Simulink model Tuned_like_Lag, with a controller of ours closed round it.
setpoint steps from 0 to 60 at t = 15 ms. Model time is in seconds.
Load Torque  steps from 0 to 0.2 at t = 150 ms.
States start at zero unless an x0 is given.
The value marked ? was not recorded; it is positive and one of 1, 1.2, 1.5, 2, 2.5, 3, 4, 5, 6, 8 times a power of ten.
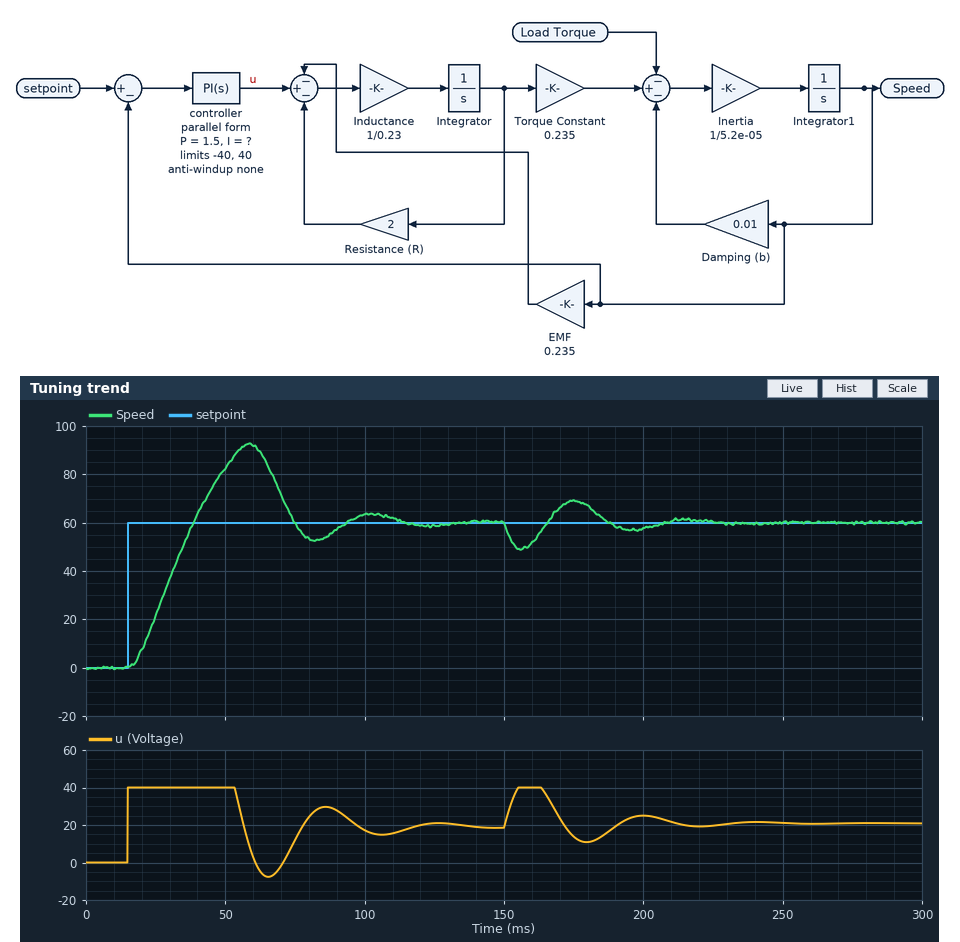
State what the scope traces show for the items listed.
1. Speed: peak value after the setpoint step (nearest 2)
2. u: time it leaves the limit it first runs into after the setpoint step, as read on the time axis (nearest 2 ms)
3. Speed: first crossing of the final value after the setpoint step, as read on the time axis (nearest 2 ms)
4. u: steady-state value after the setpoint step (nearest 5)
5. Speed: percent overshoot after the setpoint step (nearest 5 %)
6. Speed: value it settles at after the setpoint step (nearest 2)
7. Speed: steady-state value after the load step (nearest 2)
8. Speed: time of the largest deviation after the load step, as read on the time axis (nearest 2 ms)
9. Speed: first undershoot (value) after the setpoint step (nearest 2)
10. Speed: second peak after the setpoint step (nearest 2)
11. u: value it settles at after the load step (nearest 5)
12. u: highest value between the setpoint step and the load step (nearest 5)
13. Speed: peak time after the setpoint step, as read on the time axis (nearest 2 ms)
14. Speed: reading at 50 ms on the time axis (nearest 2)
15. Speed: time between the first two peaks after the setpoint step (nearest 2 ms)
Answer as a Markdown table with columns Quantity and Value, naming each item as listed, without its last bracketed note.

| Quantity | Value |
|---|---|
| Speed: peak value after the setpoint step | 92 |
| u: time it leaves the limit it first runs into after the setpoint step, as read on the time axis | 54 ms |
| Speed: first crossing of the final value after the setpoint step, as read on the time axis | 38 ms |
| u: steady-state value after the setpoint step | 20 |
| Speed: percent overshoot after the setpoint step | 55 % |
| Speed: value it settles at after the setpoint step | 60 |
| Speed: steady-state value after the load step | 60 |
| Speed: time of the largest deviation after the load step, as read on the time axis | 156 ms |
| Speed: first undershoot (value) after the setpoint step | 52 |
| Speed: second peak after the setpoint step | 64 |
| u: value it settles at after the load step | 20 |
| u: highest value between the setpoint step and the load step | 40 |
| Speed: peak time after the setpoint step, as read on the time axis | 58 ms |
| Speed: reading at 50 ms on the time axis | 82 |
| Speed: time between the first two peaks after the setpoint step | 44 ms |
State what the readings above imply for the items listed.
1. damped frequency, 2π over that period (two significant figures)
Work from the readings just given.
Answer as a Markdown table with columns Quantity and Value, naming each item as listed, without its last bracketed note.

| Quantity | Value |
|---|---|
| damped frequency, 2π over that period | 0.14 rad/ms |
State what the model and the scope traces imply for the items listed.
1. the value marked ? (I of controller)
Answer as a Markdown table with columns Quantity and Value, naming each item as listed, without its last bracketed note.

| Quantity | Value |
|---|---|
| the value marked ? | 150 |
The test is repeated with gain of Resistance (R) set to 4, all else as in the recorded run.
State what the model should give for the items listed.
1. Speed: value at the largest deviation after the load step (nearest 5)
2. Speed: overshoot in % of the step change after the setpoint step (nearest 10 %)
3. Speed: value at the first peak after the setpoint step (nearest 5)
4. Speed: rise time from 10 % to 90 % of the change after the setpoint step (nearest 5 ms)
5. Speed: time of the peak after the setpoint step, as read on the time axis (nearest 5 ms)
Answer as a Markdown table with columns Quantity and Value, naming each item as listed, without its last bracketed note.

| Quantity | Value |
|---|---|
| Speed: value at the largest deviation after the load step | 50 |
| Speed: overshoot in % of the step change after the setpoint step | 40 % |
| Speed: value at the first peak after the setpoint step | 85 |
| Speed: rise time from 10 % to 90 % of the change after the setpoint step | 20 ms |
| Speed: time of the peak after the setpoint step, as read on the time axis | 65 ms |
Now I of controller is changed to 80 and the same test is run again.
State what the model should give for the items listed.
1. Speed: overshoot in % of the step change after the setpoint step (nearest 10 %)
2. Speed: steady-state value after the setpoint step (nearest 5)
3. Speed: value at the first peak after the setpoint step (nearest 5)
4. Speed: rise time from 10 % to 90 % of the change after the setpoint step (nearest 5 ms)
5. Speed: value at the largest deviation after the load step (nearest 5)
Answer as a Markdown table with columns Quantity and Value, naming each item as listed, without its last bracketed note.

| Quantity | Value |
|---|---|
| Speed: overshoot in % of the step change after the setpoint step | 40 % |
| Speed: steady-state value after the setpoint step | 60 |
| Speed: value at the first peak after the setpoint step | 80 |
| Speed: rise time from 10 % to 90 % of the change after the setpoint step | 15 ms |
| Speed: value at the largest deviation after the load step | 50 |
